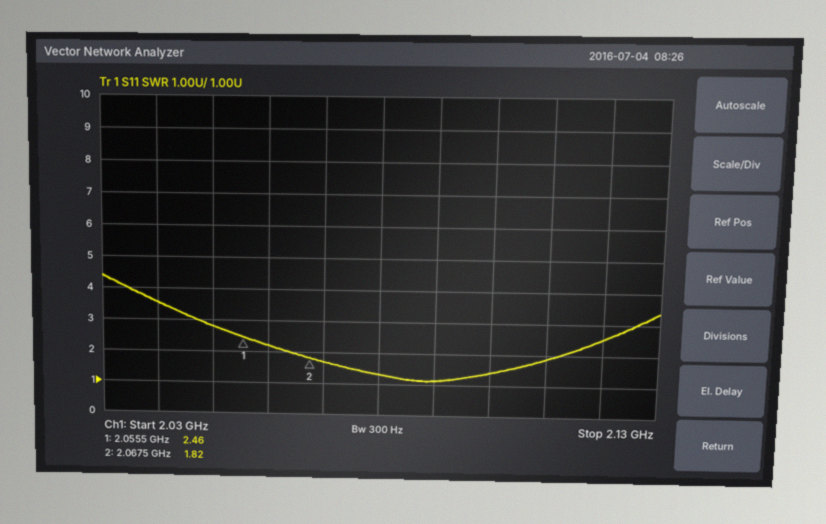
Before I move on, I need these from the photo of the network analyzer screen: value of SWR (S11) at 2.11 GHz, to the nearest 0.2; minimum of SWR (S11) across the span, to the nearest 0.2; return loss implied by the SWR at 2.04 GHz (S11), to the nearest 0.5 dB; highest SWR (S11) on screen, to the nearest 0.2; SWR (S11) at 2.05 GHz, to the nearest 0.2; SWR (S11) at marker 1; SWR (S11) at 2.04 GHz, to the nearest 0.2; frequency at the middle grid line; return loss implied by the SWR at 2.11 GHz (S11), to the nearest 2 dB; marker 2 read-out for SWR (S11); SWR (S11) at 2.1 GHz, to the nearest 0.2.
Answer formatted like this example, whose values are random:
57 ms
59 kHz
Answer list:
1.8
1.2
5.0 dB
4.4
2.8
2.46
3.6
2.08 GHz
10 dB
1.82
1.4
